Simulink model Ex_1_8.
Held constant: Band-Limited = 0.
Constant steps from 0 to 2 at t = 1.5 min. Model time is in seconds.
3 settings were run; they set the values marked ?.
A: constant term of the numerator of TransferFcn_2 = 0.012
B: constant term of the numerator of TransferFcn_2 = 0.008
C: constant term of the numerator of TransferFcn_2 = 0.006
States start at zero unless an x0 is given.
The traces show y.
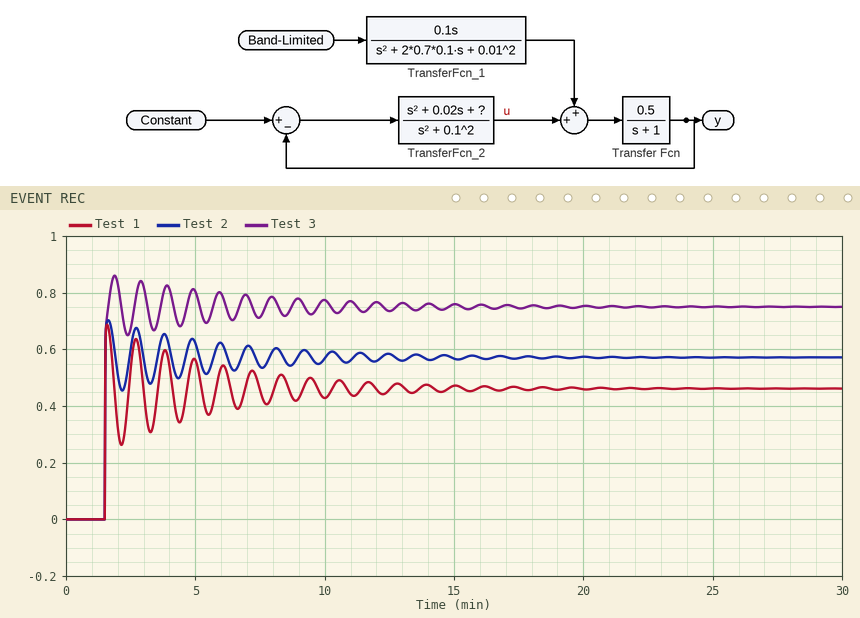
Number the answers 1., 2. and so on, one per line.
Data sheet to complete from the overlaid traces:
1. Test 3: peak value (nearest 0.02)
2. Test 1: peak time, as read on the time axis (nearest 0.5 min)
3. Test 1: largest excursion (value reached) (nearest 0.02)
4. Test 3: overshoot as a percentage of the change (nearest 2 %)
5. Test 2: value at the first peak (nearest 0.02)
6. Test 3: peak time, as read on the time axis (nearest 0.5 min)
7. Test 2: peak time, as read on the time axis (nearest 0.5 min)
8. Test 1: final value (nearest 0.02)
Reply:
1. 0.86
2. 1.5 min
3. 0.68
4. 14 %
5. 0.70
6. 2.0 min
7. 1.5 min
8. 0.46
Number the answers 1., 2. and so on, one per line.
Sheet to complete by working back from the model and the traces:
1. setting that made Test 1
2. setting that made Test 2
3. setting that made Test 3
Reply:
1. C
2. B
3. A
